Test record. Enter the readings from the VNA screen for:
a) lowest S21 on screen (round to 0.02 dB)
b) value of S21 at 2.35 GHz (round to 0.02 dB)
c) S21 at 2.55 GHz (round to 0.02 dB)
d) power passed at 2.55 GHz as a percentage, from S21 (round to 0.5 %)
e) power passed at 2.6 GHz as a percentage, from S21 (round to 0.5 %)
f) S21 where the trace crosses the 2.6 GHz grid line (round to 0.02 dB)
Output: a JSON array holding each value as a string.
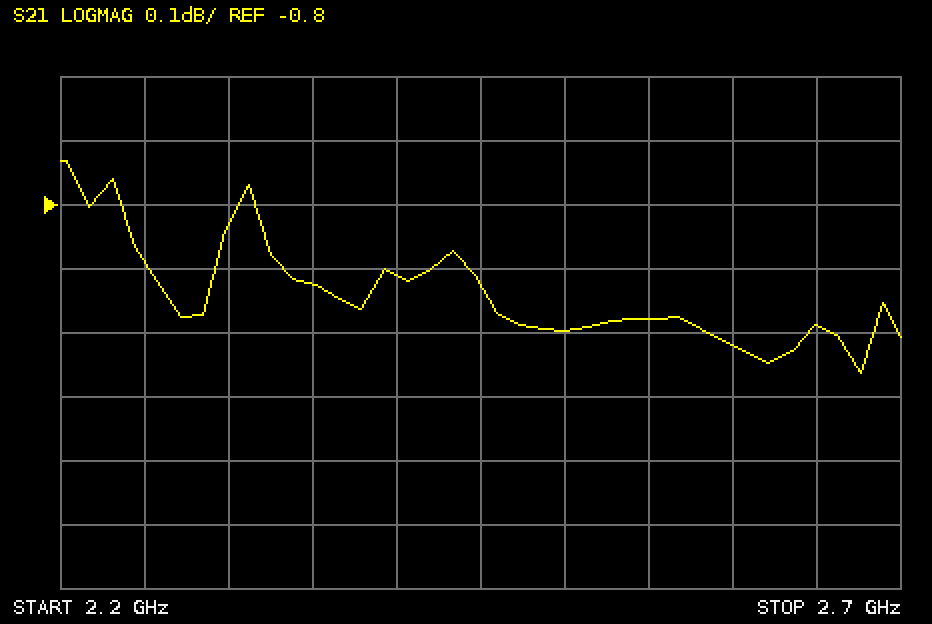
["-1.06 dB", "-0.92 dB", "-0.98 dB", "80.0 %", "79.0 %", "-1.02 dB"]
